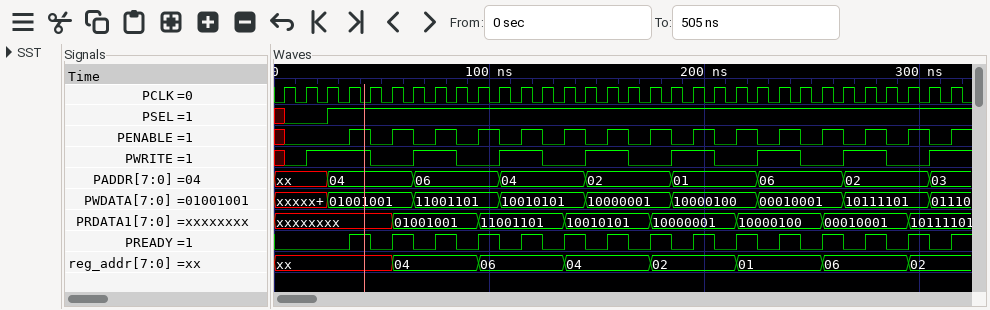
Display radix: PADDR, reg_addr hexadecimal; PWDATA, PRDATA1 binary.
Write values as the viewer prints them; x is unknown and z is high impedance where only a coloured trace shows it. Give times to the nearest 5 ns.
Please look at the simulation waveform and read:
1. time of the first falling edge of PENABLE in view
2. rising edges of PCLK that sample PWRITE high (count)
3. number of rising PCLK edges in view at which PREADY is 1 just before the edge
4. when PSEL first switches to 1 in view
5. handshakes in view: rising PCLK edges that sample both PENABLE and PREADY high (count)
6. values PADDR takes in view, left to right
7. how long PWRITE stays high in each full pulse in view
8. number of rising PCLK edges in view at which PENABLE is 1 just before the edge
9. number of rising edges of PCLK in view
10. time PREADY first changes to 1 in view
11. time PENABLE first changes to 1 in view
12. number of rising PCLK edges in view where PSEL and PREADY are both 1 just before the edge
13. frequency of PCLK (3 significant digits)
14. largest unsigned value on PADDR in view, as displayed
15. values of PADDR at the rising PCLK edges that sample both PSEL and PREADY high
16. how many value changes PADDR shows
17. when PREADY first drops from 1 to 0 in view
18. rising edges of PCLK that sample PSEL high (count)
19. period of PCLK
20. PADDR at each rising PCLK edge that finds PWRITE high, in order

45 ns
16
14
25 ns
14
xx, 04, 06, 04, 02, 01, 06, 02, 03
30 ns, 20 ns, 20 ns, 20 ns, 20 ns, 20 ns, 20 ns
14
32
35 ns
35 ns
14
100 MHz
06
04, 04, 06, 06, 04, 04, 02, 02, 01, 01, 06, 06, 02, 02
8
45 ns
29
10 ns
xx, 04, 04, 06, 06, 04, 04, 02, 02, 01, 01, 06, 06, 02, 02, 03
